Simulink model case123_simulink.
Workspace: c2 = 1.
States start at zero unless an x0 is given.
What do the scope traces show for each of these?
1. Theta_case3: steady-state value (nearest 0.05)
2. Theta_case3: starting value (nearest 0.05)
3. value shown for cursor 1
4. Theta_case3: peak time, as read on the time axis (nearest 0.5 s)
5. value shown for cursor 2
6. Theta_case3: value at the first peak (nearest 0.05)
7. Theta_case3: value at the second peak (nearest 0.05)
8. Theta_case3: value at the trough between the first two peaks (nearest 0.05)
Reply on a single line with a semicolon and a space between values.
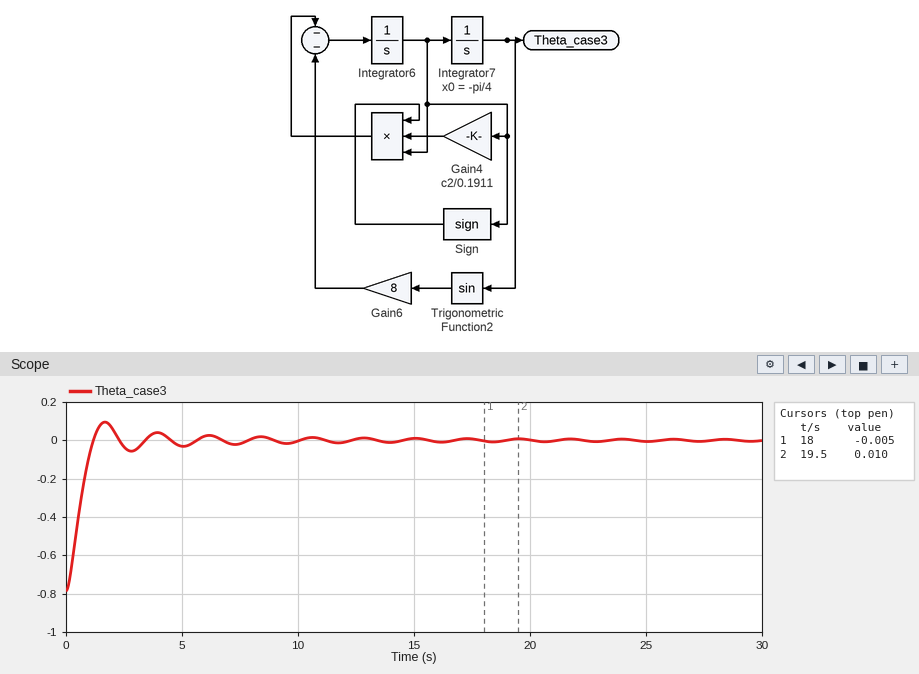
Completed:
0.00; -0.80; -0.005; 1.5 s; 0.010; 0.10; 0.05; -0.05
